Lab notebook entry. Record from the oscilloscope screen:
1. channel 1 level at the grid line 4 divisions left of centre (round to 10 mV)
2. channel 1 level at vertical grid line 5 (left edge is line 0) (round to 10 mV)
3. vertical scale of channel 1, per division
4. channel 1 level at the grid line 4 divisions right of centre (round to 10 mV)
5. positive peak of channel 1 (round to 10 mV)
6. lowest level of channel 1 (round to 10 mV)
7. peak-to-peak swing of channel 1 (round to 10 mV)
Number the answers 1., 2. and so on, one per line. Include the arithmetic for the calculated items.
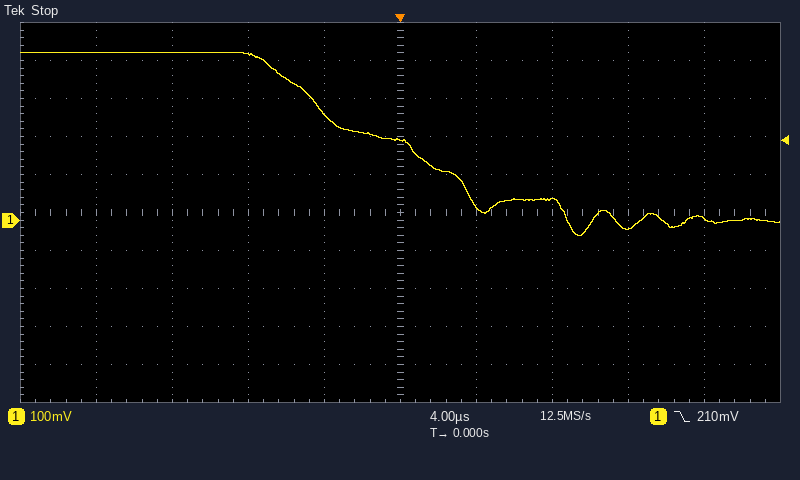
1. 440 mV
2. 210 mV
3. 100 mV
4. 0 mV
5. 440 mV
6. -40 mV
7. 440 mV − (-40 mV) = 480 mV
